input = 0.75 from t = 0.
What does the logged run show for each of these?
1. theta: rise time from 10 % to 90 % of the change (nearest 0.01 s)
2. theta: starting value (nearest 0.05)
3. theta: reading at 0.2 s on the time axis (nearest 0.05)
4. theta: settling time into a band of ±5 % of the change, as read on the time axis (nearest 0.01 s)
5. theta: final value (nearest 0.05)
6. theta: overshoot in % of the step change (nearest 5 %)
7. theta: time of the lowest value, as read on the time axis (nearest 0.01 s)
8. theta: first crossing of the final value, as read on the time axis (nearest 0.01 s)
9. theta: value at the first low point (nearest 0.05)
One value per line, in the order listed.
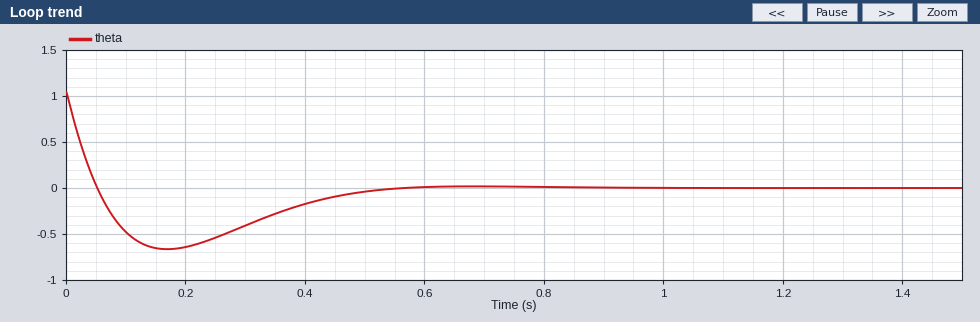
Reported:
0.04 s
1.05
-0.65
0.49 s
0.00
65 %
0.17 s
0.05 s
-0.65
